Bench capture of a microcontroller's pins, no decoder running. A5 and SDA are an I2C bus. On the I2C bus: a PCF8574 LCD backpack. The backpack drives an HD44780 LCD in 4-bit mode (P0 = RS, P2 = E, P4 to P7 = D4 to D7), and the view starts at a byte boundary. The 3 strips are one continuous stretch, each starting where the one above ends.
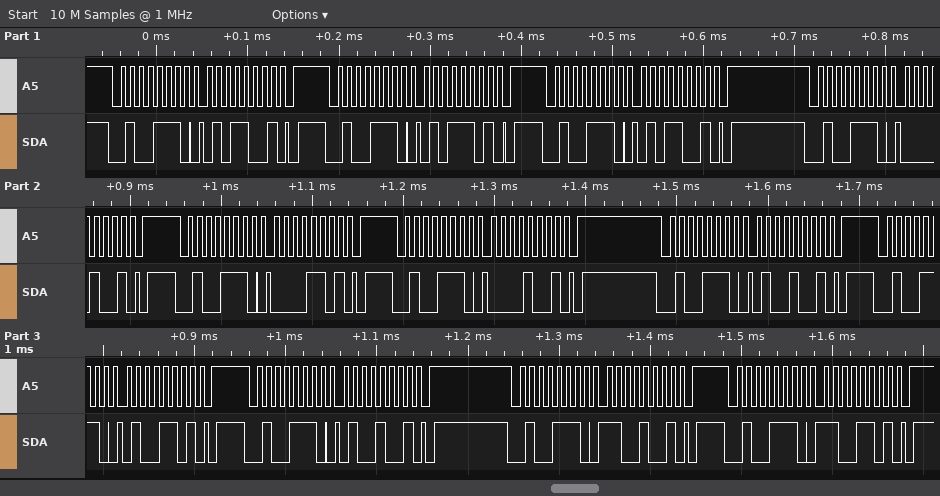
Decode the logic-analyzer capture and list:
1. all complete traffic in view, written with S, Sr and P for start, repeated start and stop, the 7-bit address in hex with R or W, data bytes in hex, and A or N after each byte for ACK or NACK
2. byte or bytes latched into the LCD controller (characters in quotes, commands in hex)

S 27W A 59 A P S 27W A 5D A P S 27W A 59 A P S 27W A 09 A P S 27W A 0D A P S 27W A 09 A P S 27W A 49 A P S 27W A 4D A P S 27W A 49 A P S 27W A C9 A P S 27W A CD A P
'P'
